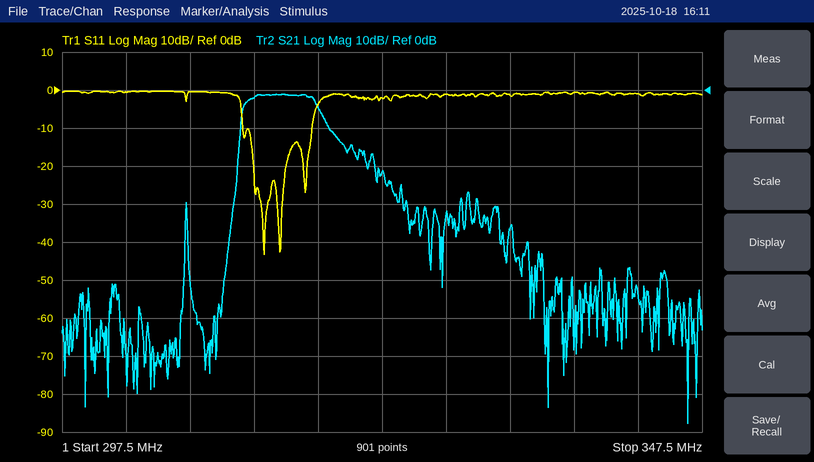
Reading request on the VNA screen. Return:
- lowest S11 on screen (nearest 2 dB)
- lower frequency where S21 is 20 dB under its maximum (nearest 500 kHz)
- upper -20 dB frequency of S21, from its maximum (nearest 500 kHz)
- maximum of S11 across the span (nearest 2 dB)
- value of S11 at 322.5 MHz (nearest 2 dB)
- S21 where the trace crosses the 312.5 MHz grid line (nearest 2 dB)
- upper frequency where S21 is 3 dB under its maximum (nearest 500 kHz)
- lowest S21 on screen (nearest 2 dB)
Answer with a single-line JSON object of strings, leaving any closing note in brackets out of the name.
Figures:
{"lowest S11 on screen": "-44 dB", "lower frequency where S21 is 20 dB under its maximum": "311.0 MHz", "upper -20 dB frequency of S21, from its maximum": "322.0 MHz", "maximum of S11 across the span": "0 dB", "value of S11 at 322.5 MHz": "-2 dB", "S21 where the trace crosses the 312.5 MHz grid line": "-2 dB", "upper frequency where S21 is 3 dB under its maximum": "317.5 MHz", "lowest S21 on screen": "-88 dB"}
